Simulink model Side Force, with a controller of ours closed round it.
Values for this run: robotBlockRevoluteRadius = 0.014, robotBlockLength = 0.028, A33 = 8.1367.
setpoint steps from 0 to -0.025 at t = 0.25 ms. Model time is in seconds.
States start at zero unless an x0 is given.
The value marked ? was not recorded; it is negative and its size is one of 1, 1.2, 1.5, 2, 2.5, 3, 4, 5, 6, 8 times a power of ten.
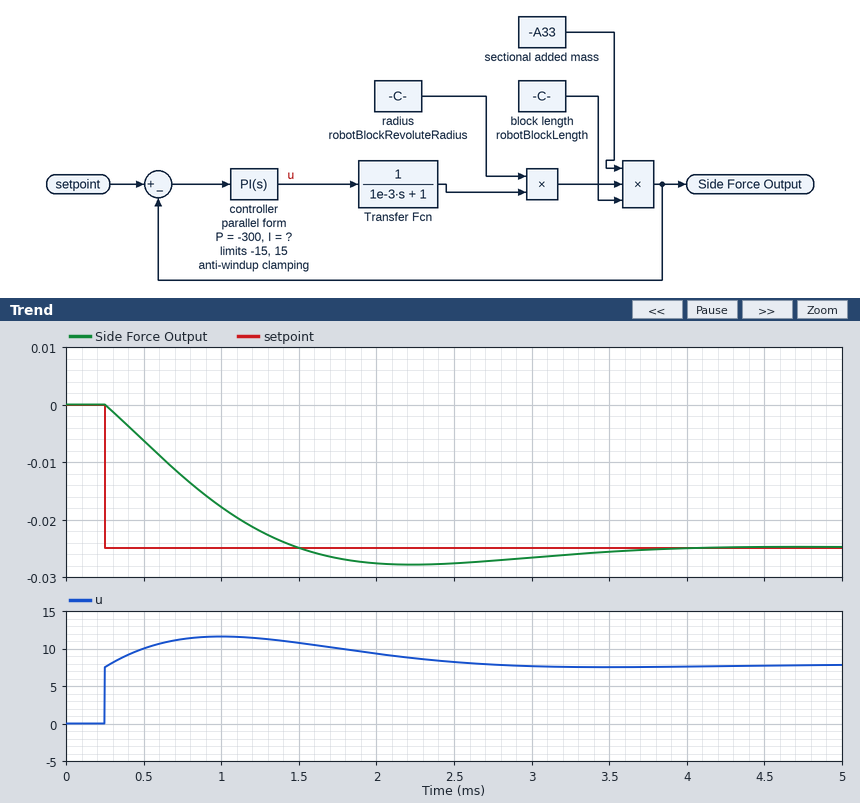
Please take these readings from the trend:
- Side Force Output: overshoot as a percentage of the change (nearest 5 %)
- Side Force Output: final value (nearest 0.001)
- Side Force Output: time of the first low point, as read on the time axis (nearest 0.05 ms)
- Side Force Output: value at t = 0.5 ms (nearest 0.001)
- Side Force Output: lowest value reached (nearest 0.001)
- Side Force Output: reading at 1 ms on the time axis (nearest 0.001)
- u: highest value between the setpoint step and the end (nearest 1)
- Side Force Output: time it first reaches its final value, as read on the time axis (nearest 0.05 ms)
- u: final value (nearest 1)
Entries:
10 %
-0.025
2.25 ms
-0.006
-0.028
-0.018
12
1.50 ms
8
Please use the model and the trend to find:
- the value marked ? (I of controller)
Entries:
-800000
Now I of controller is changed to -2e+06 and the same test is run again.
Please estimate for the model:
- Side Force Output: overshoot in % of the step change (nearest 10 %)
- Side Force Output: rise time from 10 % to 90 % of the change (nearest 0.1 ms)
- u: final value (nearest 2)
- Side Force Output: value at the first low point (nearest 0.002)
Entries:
20 %
0.6 ms
8
-0.030
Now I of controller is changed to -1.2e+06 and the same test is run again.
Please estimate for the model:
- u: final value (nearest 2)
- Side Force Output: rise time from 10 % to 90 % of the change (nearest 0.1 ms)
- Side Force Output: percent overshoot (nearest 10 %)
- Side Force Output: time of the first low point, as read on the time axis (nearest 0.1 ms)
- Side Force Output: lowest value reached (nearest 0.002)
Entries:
8
0.7 ms
20 %
1.8 ms
-0.030
